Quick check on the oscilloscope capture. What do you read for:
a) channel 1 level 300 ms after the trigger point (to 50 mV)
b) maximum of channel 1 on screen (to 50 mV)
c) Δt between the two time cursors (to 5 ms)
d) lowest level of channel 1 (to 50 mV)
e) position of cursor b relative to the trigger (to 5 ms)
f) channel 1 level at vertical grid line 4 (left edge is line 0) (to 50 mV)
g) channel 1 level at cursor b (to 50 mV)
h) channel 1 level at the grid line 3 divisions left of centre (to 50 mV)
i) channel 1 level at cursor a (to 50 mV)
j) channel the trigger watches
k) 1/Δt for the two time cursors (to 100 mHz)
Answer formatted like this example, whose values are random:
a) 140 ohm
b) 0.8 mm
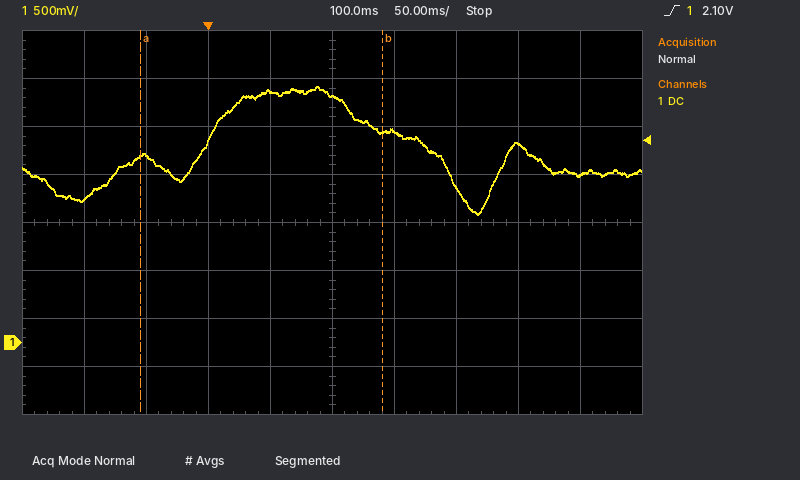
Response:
a) 1.75 V
b) 2.65 V
c) 195 ms
d) 1.35 V
e) +140 ms
f) 2.60 V
g) 2.20 V
h) 1.95 V
i) 1.95 V
j) channel 1
k) 5.1 Hz
